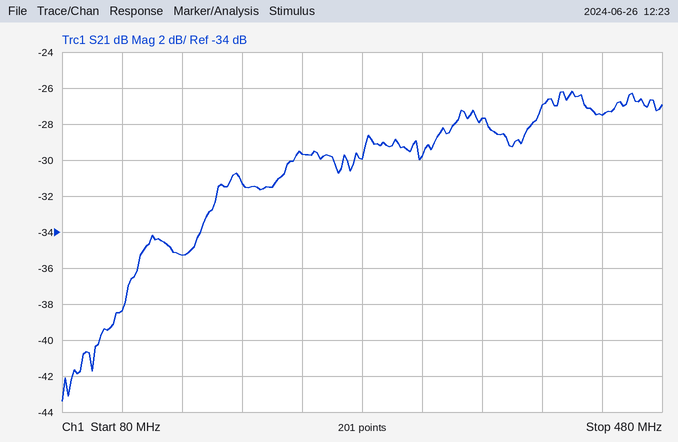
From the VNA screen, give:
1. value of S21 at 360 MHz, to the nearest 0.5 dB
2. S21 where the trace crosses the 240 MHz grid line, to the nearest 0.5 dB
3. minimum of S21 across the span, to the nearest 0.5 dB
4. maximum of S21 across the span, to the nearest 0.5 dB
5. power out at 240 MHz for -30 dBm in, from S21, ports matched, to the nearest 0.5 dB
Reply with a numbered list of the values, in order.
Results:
1. -27.5 dB
2. -29.5 dB
3. -43.5 dB
4. -26.0 dB
5. -59.5 dBm
